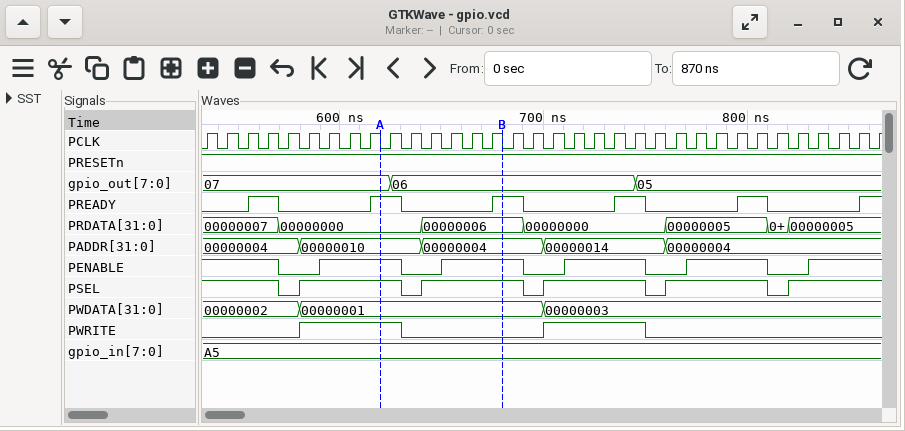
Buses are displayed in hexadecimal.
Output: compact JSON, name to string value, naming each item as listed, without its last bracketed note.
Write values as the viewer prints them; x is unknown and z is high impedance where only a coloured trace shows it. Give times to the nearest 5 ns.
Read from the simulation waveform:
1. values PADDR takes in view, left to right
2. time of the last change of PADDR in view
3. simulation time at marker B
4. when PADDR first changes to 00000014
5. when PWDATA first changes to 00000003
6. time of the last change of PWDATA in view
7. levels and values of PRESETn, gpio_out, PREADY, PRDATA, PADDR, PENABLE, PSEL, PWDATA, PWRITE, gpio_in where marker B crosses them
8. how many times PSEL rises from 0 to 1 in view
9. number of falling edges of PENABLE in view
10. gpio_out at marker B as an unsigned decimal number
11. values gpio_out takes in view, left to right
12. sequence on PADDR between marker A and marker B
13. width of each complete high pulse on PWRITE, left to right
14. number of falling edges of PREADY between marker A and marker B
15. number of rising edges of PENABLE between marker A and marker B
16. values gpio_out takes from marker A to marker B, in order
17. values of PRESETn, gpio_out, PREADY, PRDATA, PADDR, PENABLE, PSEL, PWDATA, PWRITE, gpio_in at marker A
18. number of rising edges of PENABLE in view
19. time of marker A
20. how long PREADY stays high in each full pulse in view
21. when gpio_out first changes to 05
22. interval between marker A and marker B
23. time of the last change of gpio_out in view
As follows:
{"values PADDR takes in view, left to right": "00000004, 00000010, 00000004, 00000014, 00000004", "time of the last change of PADDR in view": "760 ns", "simulation time at marker B": "680 ns", "when PADDR first changes to 00000014": "700 ns", "when PWDATA first changes to 00000003": "700 ns", "time of the last change of PWDATA in view": "700 ns", "levels and values of PRESETn, gpio_out, PREADY, PRDATA, PADDR, PENABLE, PSEL, PWDATA, PWRITE, gpio_in where marker B crosses them": "PRESETn=1, gpio_out=06, PREADY=1, PRDATA=00000006, PADDR=00000004, PENABLE=1, PSEL=1, PWDATA=00000001, PWRITE=0, gpio_in=A5", "how many times PSEL rises from 0 to 1 in view": "5", "number of falling edges of PENABLE in view": "5", "gpio_out at marker B as an unsigned decimal number": "6", "values gpio_out takes in view, left to right": "07, 06, 05", "sequence on PADDR between marker A and marker B": "00000010, 00000004", "width of each complete high pulse on PWRITE, left to right": "50 ns, 50 ns", "number of falling edges of PREADY between marker A and marker B": "1", "number of rising edges of PENABLE between marker A and marker B": "1", "values gpio_out takes from marker A to marker B, in order": "07, 06", "values of PRESETn, gpio_out, PREADY, PRDATA, PADDR, PENABLE, PSEL, PWDATA, PWRITE, gpio_in at marker A": "PRESETn=1, gpio_out=07, PREADY=1, PRDATA=00000000, PADDR=00000010, PENABLE=1, PSEL=1, PWDATA=00000001, PWRITE=1, gpio_in=A5", "number of rising edges of PENABLE in view": "5", "time of marker A": "620 ns", "how long PREADY stays high in each full pulse in view": "15 ns, 15 ns, 15 ns, 15 ns, 15 ns", "when gpio_out first changes to 05": "745 ns", "interval between marker A and marker B": "60 ns", "time of the last change of gpio_out in view": "745 ns"}
